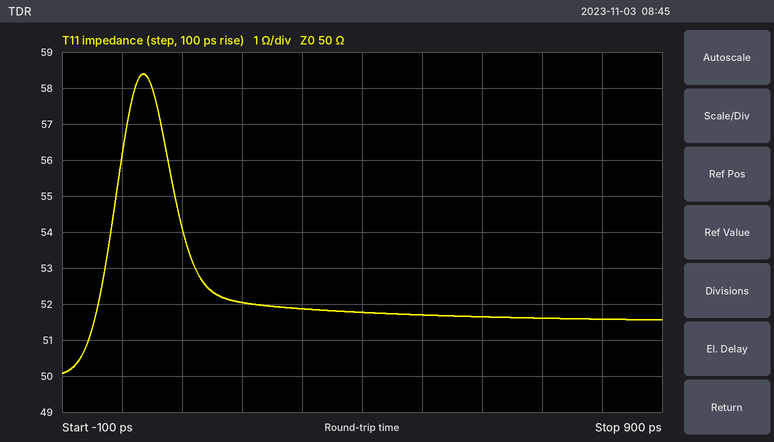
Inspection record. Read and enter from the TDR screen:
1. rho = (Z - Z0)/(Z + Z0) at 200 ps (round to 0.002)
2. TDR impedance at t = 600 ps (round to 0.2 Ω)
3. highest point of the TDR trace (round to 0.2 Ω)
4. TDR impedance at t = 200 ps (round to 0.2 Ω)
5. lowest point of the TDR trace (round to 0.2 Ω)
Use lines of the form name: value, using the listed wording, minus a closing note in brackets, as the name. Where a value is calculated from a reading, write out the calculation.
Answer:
rho = (Z - Z0)/(Z + Z0) at 200 ps: (52 − 50)/(52 + 50) ≈ +0.020
TDR impedance at t = 600 ps: 51.6 Ω
highest point of the TDR trace: 58.4 Ω
TDR impedance at t = 200 ps: 52.0 Ω
lowest point of the TDR trace: 50.0 Ω
